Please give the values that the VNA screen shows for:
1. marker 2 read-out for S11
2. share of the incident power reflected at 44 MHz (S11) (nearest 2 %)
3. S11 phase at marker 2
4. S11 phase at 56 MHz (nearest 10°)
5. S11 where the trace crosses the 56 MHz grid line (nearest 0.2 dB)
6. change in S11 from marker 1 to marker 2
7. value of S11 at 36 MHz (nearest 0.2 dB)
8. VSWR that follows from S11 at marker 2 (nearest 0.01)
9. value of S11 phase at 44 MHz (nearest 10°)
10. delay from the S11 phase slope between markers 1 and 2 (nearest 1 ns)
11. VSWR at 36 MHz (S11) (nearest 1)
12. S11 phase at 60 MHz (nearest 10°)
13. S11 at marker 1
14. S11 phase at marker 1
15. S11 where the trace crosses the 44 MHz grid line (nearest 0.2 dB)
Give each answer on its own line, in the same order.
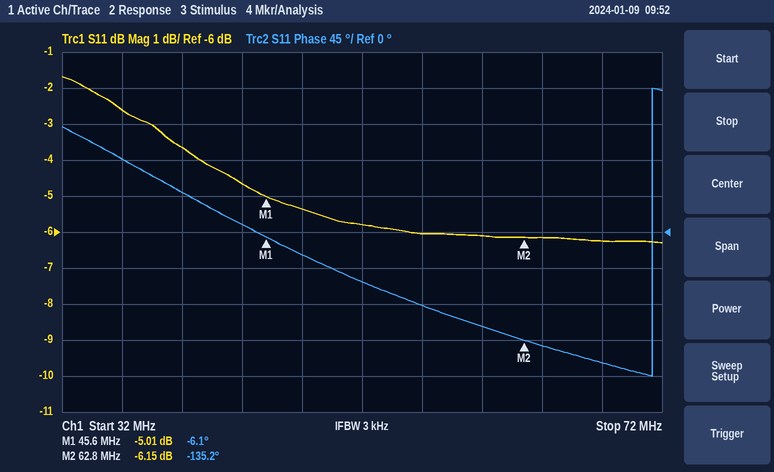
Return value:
-6.15 dB
34 %
-135.2°
-90°
-6.0 dB
-1.14 dB
-2.6 dB
2.94
10°
21 ns
7
-120°
-5.01 dB
-6.1°
-4.6 dB
